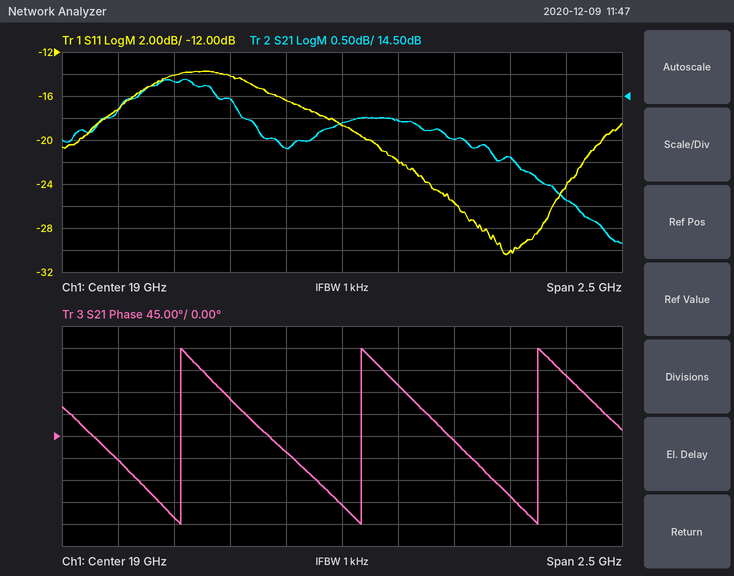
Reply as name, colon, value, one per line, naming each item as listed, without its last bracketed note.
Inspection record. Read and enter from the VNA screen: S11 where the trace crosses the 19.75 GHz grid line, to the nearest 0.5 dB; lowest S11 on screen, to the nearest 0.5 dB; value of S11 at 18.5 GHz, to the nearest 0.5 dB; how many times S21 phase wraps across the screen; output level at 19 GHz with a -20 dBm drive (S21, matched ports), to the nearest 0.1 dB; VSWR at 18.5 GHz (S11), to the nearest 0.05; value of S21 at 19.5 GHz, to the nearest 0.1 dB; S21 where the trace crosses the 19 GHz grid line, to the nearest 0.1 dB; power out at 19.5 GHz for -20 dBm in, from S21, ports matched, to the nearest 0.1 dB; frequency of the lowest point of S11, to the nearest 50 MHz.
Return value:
S11 where the trace crosses the 19.75 GHz grid line, to the nearest 0.5 dB: -30.0 dB
lowest S11 on screen, to the nearest 0.5 dB: -30.5 dB
value of S11 at 18.5 GHz, to the nearest 0.5 dB: -14.0 dB
how many times S21 phase wraps across the screen: 3
output level at 19 GHz with a -20 dBm drive (S21, matched ports), to the nearest 0.1 dB: -6.1 dBm
VSWR at 18.5 GHz (S11), to the nearest 0.05: 1.50
value of S21 at 19.5 GHz, to the nearest 0.1 dB: 13.5 dB
S21 where the trace crosses the 19 GHz grid line, to the nearest 0.1 dB: 13.9 dB
power out at 19.5 GHz for -20 dBm in, from S21, ports matched, to the nearest 0.1 dB: -6.5 dBm
frequency of the lowest point of S11, to the nearest 50 MHz: 19.75 GHz
